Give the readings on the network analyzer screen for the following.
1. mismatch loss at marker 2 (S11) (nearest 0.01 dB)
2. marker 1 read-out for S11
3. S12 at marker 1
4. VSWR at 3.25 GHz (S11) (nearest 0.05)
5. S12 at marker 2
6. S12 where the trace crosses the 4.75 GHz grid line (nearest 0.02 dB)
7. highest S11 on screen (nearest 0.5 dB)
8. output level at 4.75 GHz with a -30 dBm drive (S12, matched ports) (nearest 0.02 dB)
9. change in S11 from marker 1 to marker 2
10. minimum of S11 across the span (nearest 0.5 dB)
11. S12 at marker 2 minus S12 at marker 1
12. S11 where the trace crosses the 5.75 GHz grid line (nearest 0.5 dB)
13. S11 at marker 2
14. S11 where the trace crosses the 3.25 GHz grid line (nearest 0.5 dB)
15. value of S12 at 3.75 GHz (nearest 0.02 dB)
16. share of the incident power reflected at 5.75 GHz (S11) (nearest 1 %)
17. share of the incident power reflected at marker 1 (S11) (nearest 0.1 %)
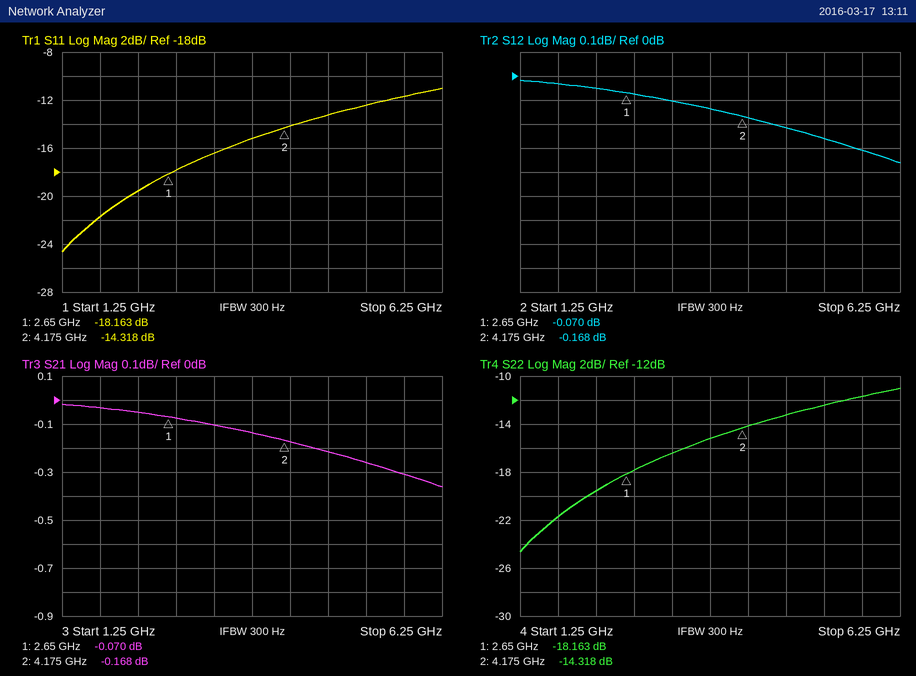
0.16 dB
-18.163 dB
-0.070 dB
1.35
-0.168 dB
-0.22 dB
-11.0 dB
-30.22 dBm
3.845 dB
-24.5 dB
-0.098 dB
-11.5 dB
-14.318 dB
-16.5 dB
-0.14 dB
7 %
1.5 %
